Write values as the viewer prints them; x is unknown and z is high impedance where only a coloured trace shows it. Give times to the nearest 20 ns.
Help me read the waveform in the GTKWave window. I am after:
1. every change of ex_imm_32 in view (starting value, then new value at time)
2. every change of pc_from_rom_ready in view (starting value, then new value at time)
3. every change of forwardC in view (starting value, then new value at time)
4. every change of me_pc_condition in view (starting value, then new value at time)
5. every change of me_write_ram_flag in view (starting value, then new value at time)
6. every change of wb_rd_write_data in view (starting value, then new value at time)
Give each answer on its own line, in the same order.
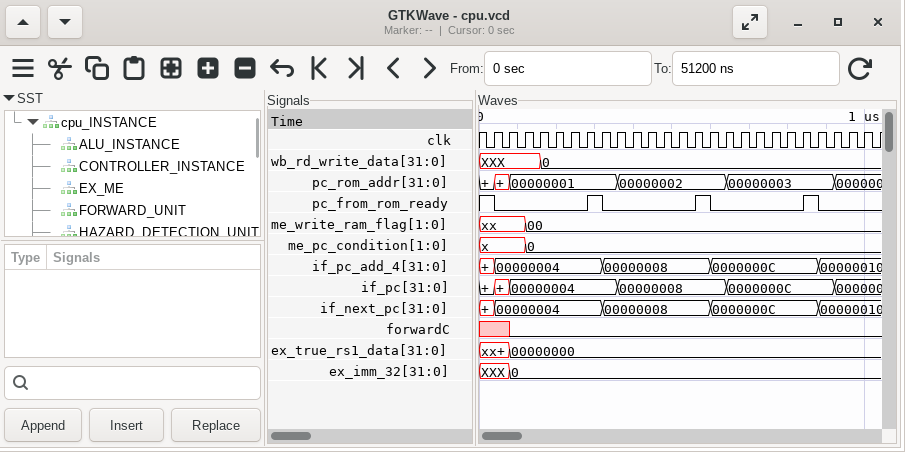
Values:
XXX, 0 at 80 ns
1, 0 at 40 ns, 1 at 280 ns, 0 at 320 ns, 1 at 560 ns, 0 at 600 ns, 1 at 840 ns, 0 at 880 ns
x, 0 at 80 ns
x, 0 at 120 ns
xx, 00 at 120 ns
XXX, 0 at 160 ns
